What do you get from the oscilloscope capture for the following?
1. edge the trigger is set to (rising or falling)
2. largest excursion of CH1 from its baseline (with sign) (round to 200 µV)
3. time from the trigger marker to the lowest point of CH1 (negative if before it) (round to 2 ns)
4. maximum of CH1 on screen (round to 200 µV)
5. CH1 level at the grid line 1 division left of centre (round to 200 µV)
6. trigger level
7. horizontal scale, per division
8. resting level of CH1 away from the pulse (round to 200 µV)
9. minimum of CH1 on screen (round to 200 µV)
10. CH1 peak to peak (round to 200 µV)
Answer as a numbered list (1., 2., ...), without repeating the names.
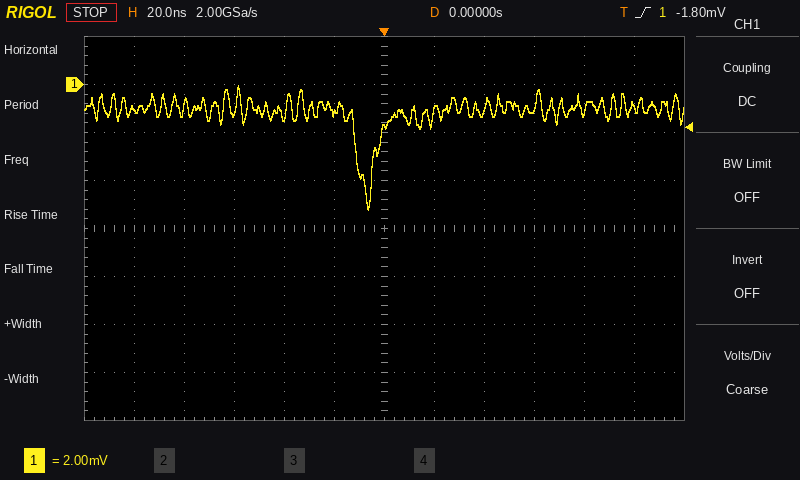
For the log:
1. rising
2. -4.2 mV
3. -6 ns
4. 0.0 mV
5. -1.2 mV
6. -1.80 mV
7. 20 ns
8. -1.0 mV
9. -5.2 mV
10. 5.2 mV
